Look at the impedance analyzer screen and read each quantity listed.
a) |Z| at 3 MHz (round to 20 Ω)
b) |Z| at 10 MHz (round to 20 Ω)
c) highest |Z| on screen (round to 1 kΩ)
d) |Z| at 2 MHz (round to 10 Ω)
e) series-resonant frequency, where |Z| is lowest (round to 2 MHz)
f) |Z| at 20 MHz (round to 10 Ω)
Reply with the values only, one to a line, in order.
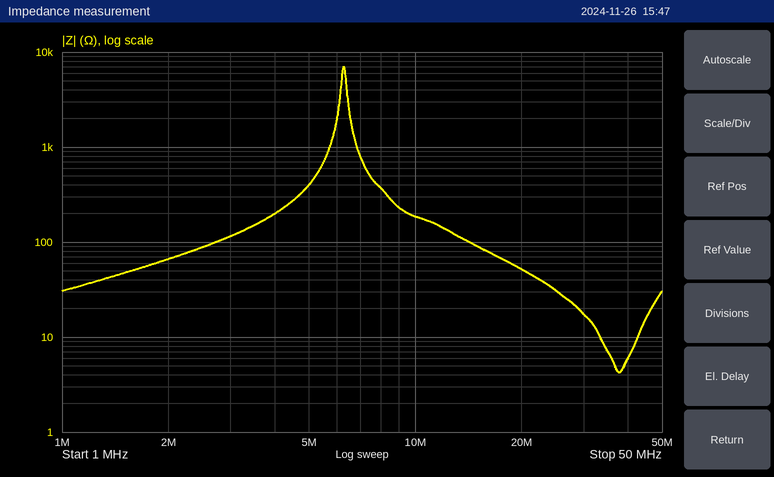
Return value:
120 Ω
180 Ω
7 kΩ
70 Ω
38 MHz
50 Ω
